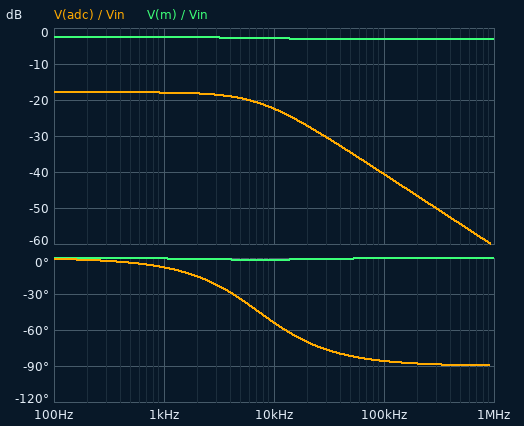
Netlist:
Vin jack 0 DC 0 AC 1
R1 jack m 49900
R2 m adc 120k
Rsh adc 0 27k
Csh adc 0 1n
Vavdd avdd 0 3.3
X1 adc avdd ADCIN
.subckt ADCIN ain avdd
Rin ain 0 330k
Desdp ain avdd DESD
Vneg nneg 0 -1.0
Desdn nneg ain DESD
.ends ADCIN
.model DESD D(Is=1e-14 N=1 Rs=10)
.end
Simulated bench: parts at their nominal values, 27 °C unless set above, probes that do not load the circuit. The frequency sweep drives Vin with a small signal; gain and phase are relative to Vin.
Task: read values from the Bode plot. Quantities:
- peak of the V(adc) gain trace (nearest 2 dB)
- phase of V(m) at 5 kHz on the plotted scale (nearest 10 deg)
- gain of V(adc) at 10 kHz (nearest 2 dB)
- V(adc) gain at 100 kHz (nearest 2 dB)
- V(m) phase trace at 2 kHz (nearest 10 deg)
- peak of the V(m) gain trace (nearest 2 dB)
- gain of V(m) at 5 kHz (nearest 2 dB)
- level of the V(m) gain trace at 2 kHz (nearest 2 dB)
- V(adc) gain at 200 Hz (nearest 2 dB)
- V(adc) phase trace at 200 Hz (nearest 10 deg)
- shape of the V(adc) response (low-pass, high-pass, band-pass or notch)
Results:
-18 dB
0 deg
-22 dB
-40 dB
0 deg
-2 dB
-2 dB
-2 dB
-18 dB
0 deg
low-pass
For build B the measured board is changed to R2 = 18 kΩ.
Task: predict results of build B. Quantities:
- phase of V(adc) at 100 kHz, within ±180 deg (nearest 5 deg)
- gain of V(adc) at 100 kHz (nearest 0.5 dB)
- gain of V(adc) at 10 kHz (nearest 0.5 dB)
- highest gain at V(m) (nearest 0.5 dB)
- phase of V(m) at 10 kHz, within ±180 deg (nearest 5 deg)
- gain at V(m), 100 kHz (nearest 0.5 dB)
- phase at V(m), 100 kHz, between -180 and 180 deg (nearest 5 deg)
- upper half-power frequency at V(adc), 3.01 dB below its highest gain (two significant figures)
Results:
-85 deg
-32.5 dB
-15.0 dB
-6.5 dB
-15 deg
-11.5 dB
-5 deg
8.7 kHz
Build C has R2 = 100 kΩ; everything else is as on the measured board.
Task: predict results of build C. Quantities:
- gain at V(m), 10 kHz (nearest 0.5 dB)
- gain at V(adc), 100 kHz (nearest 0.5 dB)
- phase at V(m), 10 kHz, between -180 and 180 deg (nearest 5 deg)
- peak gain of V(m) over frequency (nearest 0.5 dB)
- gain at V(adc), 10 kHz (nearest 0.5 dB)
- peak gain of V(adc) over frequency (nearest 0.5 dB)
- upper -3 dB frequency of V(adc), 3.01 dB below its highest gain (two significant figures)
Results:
-3.5 dB
-39.5 dB
0 deg
-3.0 dB
-21.5 dB
-17.0 dB
7.4 kHz
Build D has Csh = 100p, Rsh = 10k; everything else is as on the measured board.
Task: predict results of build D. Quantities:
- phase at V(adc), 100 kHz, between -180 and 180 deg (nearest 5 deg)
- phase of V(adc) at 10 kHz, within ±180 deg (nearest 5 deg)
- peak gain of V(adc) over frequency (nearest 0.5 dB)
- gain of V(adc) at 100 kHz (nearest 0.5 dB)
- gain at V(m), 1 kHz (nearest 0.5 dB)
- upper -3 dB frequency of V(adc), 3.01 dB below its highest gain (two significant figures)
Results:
-30 deg
-5 deg
-25.5 dB
-26.5 dB
-3.0 dB
170 kHz
